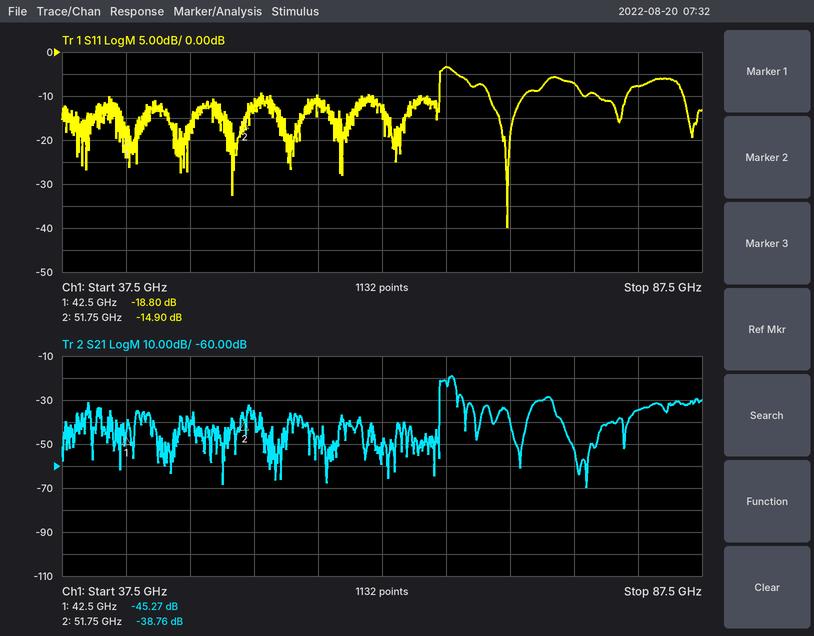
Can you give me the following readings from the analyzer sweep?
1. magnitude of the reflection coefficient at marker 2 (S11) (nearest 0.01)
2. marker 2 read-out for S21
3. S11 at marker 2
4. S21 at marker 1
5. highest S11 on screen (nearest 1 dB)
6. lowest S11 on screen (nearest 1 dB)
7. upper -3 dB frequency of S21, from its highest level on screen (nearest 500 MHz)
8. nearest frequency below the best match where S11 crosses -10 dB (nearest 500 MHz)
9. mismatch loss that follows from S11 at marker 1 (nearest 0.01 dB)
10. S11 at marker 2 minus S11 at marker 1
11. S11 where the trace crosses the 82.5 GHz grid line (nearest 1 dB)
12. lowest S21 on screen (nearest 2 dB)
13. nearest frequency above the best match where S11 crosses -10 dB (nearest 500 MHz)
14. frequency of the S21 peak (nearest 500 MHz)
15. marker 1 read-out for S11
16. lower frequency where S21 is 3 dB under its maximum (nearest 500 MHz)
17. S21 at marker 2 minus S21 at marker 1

0.18
-38.76 dB
-14.90 dB
-45.27 dB
-3 dB
-40 dB
68.0 GHz
71.0 GHz
0.06 dB
3.90 dB
-8 dB
-70 dB
73.5 GHz
68.0 GHz
-18.80 dB
67.5 GHz
6.51 dB
